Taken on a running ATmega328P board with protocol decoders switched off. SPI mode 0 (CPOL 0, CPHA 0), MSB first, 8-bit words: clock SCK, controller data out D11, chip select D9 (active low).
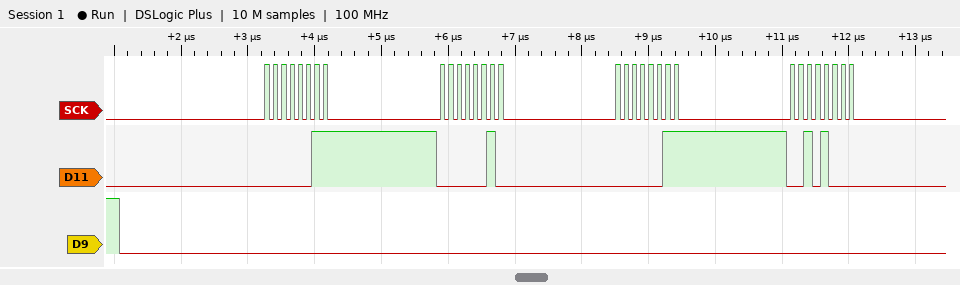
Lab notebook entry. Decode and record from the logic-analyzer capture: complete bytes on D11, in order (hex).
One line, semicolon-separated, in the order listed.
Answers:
03 02 03 28
